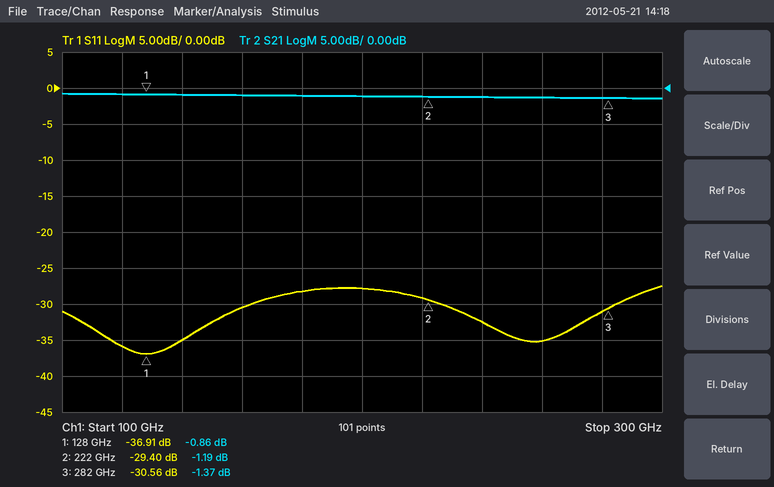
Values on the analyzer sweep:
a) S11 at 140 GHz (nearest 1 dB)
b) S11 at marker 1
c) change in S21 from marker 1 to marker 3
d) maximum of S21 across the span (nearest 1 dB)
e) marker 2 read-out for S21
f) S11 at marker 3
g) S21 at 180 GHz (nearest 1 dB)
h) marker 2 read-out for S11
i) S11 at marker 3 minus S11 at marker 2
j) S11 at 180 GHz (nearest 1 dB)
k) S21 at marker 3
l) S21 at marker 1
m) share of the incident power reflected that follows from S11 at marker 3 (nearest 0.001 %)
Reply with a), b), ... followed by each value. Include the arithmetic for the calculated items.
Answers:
a) -35 dB
b) -36.91 dB
c) -1.37 − (-0.86) = -0.51 dB
d) -1 dB
e) -1.19 dB
f) -30.56 dB
g) -1 dB
h) -29.40 dB
i) -30.56 − (-29.4) = -1.16 dB
j) -28 dB
k) -1.37 dB
l) -0.86 dB
m) 10^(-30.56/10) ≈ 0.088 %
